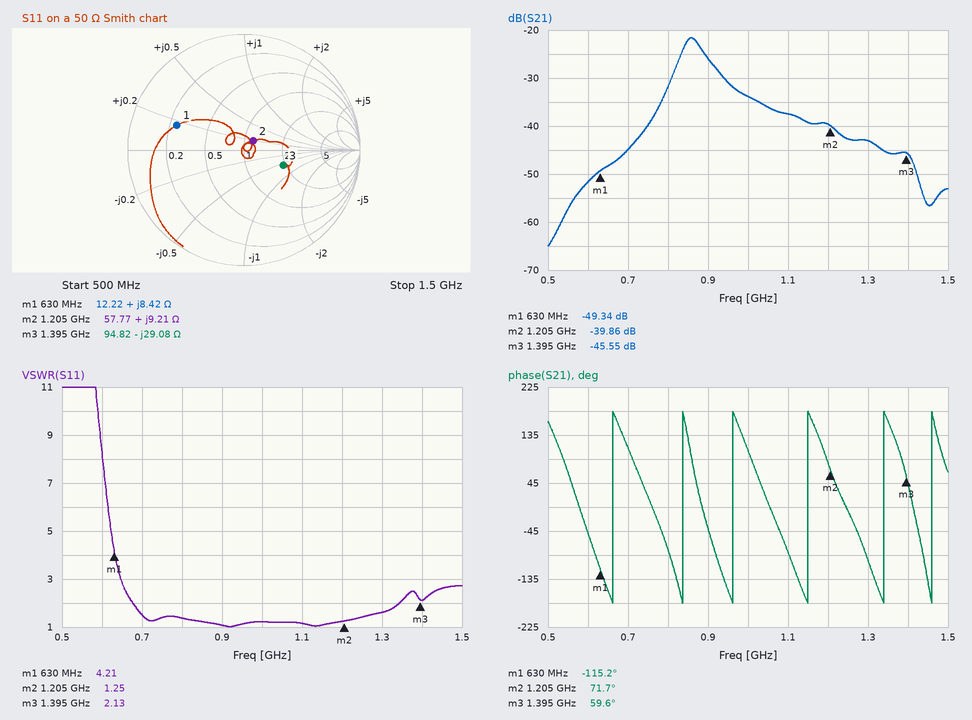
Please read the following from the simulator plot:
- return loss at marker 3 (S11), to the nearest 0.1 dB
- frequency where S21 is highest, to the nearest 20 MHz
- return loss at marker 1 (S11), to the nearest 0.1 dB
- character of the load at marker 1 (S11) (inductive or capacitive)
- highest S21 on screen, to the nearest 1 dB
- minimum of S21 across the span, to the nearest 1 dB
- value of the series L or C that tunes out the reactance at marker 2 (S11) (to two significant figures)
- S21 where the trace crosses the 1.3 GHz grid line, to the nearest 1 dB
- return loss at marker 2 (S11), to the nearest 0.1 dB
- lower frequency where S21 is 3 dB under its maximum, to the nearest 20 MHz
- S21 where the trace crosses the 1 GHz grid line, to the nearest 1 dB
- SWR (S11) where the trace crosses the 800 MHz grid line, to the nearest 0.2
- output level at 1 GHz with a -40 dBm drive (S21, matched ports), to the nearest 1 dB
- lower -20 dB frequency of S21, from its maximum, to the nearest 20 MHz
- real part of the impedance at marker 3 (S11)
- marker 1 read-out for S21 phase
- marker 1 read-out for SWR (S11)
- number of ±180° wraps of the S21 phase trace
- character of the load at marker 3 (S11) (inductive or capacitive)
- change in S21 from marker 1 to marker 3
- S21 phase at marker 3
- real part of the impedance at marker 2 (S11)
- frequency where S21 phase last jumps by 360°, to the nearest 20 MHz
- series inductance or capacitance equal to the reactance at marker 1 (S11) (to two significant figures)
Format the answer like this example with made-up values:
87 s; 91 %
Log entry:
8.8 dB; 860 MHz; 4.2 dB; inductive; -22 dB; -65 dB; 14 pF; -43 dB; 19.1 dB; 840 MHz; -34 dB; 1.4; -74 dBm; 740 MHz; 94.82 Ω; -115.2°; 4.21; 6; capacitive; 3.79 dB; 59.6°; 57.77 Ω; 1.46 GHz; 2.1 nH
